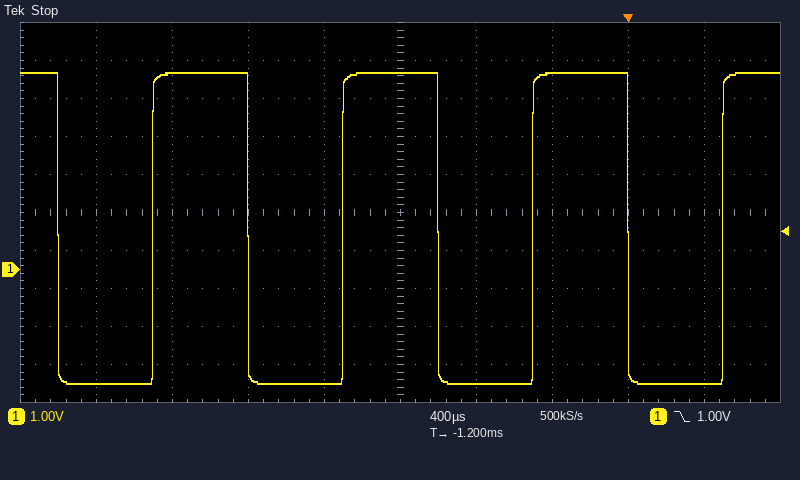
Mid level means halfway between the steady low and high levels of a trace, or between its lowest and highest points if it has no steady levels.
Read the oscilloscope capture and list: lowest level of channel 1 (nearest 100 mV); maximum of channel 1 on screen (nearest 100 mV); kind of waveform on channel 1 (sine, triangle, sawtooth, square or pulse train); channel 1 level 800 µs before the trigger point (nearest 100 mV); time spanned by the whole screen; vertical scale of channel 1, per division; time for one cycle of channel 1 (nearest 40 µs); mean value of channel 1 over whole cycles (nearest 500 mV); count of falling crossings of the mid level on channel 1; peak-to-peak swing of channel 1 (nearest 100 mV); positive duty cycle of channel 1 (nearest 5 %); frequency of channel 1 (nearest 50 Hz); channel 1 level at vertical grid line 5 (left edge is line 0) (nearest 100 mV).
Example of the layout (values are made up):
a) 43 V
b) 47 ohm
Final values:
a) -3.0 V
b) 5.2 V
c) square
d) -3.0 V
e) 4 ms
f) 1 V
g) 1.00 ms
h) 1.0 V
i) 4
j) 8.2 V
k) 50 %
l) 1.00 kHz
m) 5.2 V
